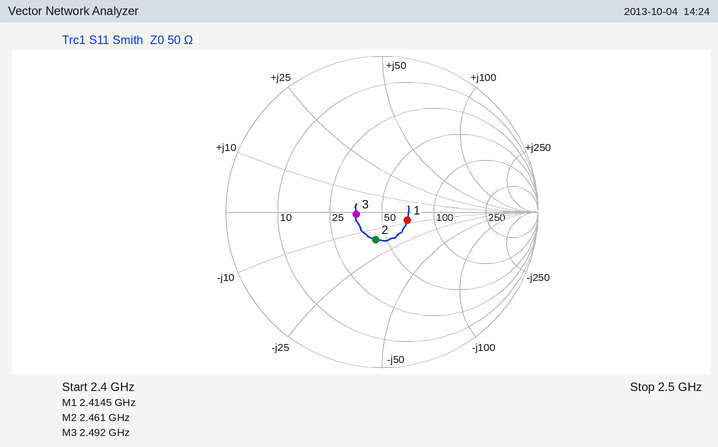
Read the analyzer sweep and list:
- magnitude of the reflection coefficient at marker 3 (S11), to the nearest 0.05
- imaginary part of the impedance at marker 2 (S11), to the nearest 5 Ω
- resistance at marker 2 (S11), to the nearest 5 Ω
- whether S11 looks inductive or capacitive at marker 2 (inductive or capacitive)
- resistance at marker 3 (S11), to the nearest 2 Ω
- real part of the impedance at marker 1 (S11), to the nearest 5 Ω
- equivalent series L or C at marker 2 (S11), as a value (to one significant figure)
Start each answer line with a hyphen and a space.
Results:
- 0.15
- -15 Ω
- 45 Ω
- capacitive
- 36 Ω
- 70 Ω
- 4 pF
